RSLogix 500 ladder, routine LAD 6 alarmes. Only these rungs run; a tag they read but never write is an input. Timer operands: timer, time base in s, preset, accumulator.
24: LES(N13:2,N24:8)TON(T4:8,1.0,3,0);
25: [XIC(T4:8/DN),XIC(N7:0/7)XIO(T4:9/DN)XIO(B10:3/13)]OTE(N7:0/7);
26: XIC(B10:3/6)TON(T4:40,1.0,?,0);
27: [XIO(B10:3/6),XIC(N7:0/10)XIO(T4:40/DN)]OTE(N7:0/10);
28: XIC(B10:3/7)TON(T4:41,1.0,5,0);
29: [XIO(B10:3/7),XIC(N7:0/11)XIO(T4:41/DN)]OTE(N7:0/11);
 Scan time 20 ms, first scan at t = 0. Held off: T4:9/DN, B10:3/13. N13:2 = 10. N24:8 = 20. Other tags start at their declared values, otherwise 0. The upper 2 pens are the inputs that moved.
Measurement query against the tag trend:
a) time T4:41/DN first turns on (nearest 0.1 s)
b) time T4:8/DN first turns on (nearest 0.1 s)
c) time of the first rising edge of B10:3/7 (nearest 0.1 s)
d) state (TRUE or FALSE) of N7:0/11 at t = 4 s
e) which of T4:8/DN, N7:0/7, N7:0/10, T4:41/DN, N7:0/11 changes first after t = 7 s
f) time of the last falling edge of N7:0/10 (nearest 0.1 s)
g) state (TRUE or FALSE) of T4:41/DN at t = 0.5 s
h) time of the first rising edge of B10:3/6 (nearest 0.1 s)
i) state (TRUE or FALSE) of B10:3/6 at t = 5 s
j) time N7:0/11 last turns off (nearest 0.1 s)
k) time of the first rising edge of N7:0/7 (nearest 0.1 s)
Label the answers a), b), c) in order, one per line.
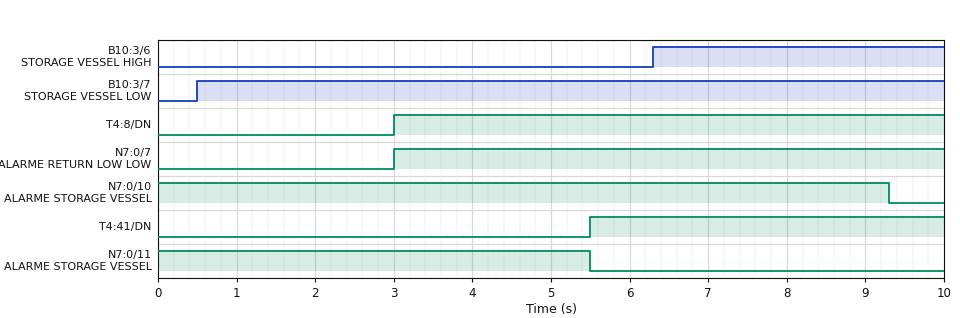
a) 5.5 s
b) 3.0 s
c) 0.5 s
d) TRUE
e) N7:0/10
f) 9.3 s
g) FALSE
h) 6.3 s
i) FALSE
j) 5.5 s
k) 3.0 s
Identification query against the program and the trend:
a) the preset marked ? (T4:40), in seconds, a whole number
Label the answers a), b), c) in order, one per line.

a) 3 s
